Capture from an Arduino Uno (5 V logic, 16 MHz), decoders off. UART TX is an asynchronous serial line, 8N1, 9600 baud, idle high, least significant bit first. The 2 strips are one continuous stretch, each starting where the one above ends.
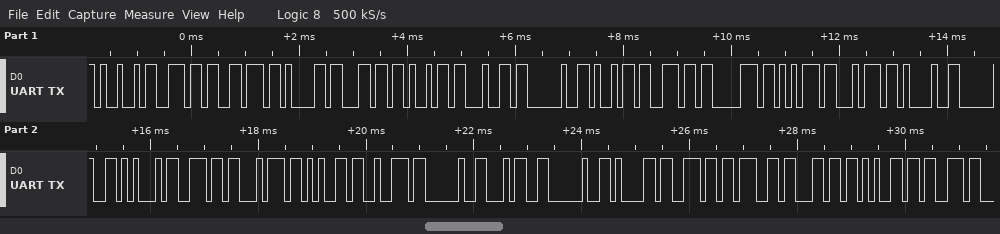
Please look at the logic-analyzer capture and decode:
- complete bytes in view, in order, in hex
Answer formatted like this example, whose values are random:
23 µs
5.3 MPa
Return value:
49 6E 76 61 6C 69 64 20 69 6E 70 75 74 21 20 45 6E 74 65 72 20 34 20 61 6E 67 6C 65 73
